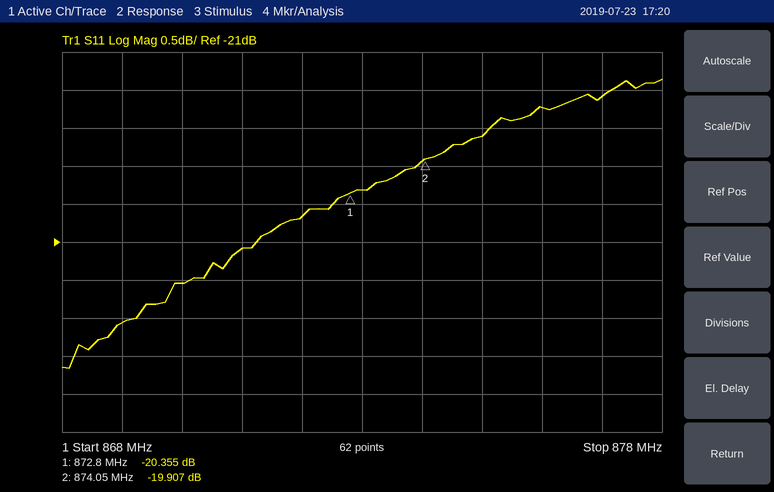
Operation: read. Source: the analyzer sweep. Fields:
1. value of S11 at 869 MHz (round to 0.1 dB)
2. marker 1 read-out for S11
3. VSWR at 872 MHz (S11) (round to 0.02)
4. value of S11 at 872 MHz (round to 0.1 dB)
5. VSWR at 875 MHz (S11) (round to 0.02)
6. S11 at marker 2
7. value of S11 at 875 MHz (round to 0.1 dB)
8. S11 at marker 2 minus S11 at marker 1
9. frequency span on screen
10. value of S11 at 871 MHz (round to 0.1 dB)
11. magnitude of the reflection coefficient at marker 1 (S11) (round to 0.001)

-22.1 dB
-20.355 dB
1.20
-20.7 dB
1.24
-19.907 dB
-19.6 dB
0.448 dB
10 MHz
-21.1 dB
0.096
